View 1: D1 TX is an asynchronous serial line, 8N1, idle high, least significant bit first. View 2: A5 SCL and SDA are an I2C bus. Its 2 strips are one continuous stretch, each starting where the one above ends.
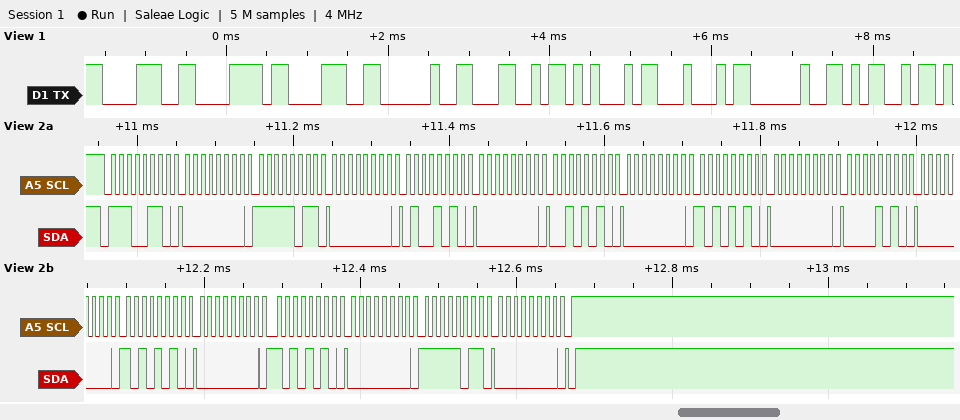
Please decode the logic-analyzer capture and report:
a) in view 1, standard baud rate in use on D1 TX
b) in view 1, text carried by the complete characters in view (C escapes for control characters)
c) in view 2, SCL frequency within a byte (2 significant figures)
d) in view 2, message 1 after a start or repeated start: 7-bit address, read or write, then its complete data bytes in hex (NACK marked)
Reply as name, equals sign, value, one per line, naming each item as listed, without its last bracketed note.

in view 1, standard baud rate in use on D1 TX = 9600 baud
in view 1, text carried by the complete characters in view = "8x8 LED M"
in view 2, SCL frequency within a byte = 100 kHz
in view 2, message 1 after a start or repeated start: 7-bit address, read or write, then its complete data bytes in hex = 0x73 write: 00 FB 00 4A 00 2A 00 AA 00 0A 00 AA 00 AA 00 FB 00
